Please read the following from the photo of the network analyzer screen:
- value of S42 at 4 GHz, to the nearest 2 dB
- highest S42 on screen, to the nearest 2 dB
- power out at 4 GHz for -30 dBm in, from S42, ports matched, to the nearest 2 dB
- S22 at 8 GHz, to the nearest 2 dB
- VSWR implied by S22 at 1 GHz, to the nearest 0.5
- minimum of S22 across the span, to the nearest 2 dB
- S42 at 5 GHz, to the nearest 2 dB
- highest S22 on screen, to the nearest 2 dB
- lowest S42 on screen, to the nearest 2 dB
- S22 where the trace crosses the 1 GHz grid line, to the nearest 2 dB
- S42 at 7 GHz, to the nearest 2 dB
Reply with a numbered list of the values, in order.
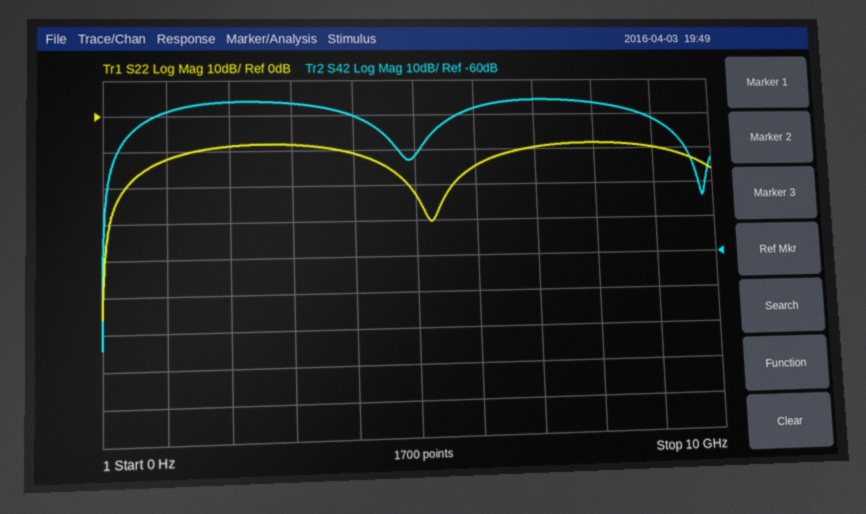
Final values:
1. -20 dB
2. -16 dB
3. -50 dBm
4. -8 dB
5. 1.5
6. -56 dB
7. -32 dB
8. -8 dB
9. -84 dB
10. -12 dB
11. -16 dB
